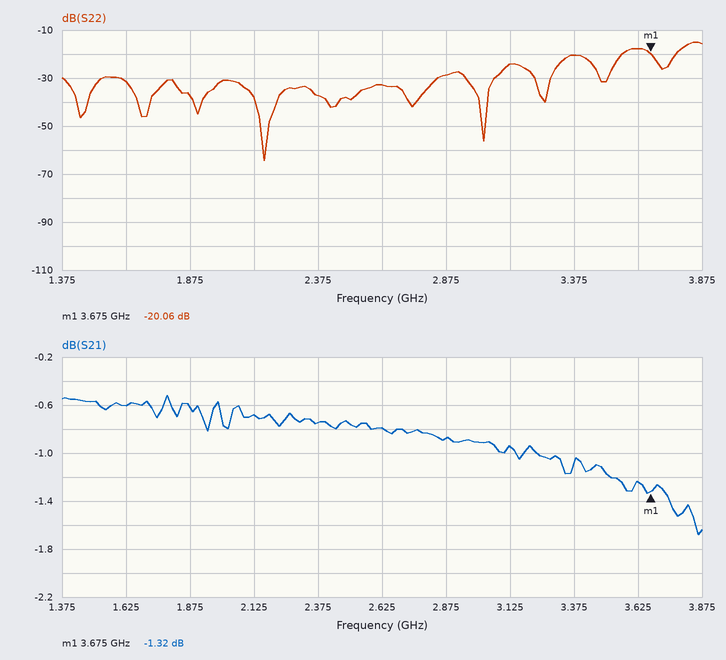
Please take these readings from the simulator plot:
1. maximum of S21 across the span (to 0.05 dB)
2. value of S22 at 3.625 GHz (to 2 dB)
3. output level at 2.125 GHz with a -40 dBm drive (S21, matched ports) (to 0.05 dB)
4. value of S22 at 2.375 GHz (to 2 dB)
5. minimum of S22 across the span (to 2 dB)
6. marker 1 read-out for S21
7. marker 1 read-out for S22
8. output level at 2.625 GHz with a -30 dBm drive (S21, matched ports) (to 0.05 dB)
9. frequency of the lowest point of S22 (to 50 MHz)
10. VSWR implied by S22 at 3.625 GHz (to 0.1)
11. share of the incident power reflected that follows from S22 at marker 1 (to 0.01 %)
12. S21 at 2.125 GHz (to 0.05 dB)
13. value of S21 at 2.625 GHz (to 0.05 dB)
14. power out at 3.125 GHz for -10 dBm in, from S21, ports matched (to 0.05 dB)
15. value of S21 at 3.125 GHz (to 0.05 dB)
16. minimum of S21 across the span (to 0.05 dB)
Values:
-0.50 dB
-18 dB
-40.70 dBm
-38 dB
-64 dB
-1.32 dB
-20.06 dB
-30.80 dBm
2.15 GHz
1.3
0.99 %
-0.70 dB
-0.80 dB
-10.95 dBm
-0.95 dB
-1.70 dB
